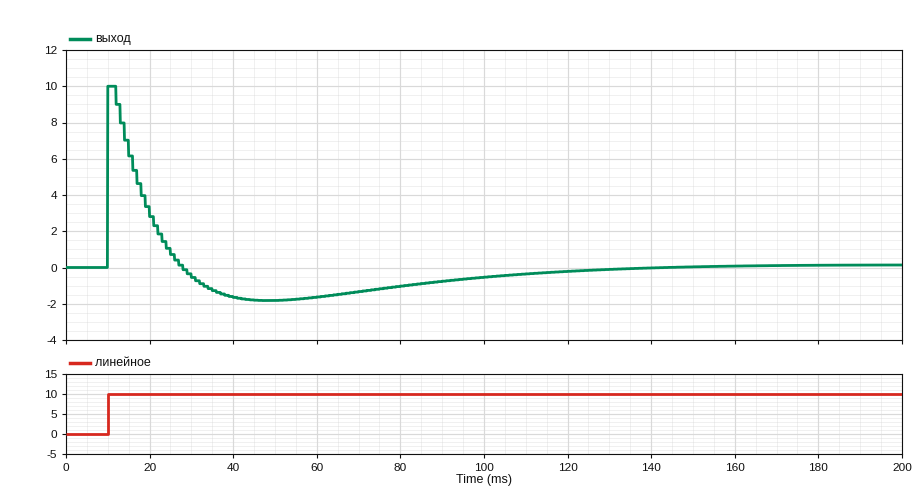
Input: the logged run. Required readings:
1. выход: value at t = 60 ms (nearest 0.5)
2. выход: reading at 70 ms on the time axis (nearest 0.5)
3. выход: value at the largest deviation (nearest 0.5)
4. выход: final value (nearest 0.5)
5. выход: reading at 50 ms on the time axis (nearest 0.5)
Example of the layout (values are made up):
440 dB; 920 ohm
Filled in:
-1.5; -1.5; 10.0; 0.0; -2.0
